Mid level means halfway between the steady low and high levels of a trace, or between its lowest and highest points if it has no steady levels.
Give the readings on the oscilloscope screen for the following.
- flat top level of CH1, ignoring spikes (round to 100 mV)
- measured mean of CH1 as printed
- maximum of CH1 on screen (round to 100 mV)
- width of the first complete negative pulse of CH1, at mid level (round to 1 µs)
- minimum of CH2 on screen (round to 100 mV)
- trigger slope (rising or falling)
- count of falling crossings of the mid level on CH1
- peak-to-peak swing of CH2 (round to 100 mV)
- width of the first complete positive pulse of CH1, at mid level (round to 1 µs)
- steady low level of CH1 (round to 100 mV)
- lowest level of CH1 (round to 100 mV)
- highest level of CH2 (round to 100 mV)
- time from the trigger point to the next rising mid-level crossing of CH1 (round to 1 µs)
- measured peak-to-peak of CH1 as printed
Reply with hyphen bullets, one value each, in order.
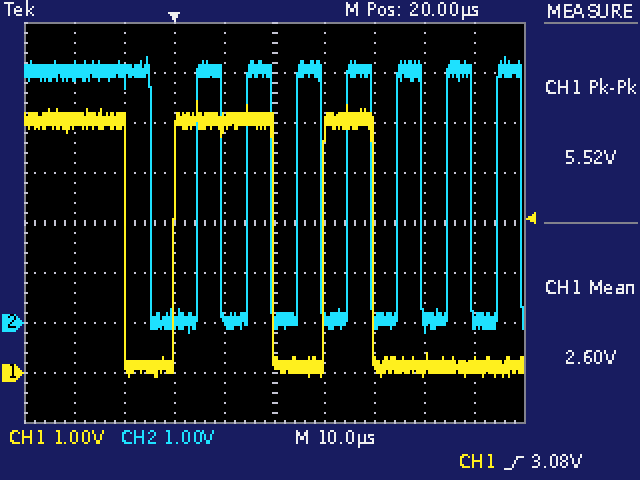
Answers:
- 5.0 V
- 2.60 V
- 5.4 V
- 10 µs
- -200 mV
- rising
- 3
- 5.5 V
- 20 µs
- 100 mV
- -100 mV
- 5.3 V
- 30 µs
- 5.52 V
